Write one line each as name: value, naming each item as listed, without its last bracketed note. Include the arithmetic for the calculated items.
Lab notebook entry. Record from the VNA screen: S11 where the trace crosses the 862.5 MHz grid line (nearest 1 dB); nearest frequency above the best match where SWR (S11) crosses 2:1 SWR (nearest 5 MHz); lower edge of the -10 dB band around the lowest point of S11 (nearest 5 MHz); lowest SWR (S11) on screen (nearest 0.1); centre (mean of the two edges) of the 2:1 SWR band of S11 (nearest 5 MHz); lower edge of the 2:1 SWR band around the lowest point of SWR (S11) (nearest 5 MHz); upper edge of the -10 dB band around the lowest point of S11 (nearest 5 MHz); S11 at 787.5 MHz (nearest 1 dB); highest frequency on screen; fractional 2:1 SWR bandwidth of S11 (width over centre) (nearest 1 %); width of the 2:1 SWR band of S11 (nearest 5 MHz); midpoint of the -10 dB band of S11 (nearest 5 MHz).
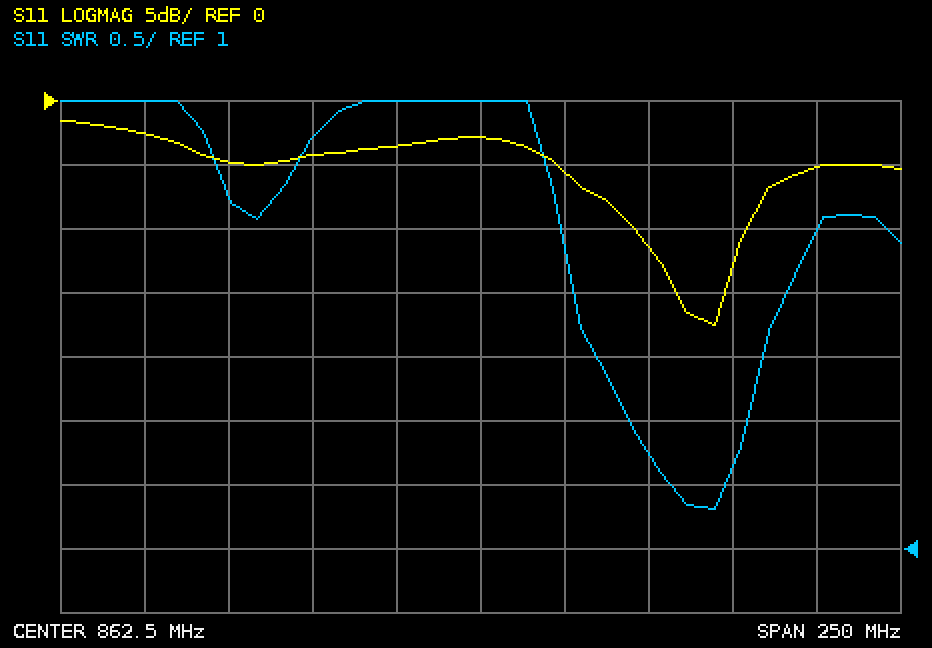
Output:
S11 where the trace crosses the 862.5 MHz grid line: -3 dB
nearest frequency above the best match where SWR (S11) crosses 2:1 SWR: 940 MHz
lower edge of the -10 dB band around the lowest point of S11: 910 MHz
lowest SWR (S11) on screen: 1.3
centre (mean of the two edges) of the 2:1 SWR band of S11: 925 MHz
lower edge of the 2:1 SWR band around the lowest point of SWR (S11): 905 MHz
upper edge of the -10 dB band around the lowest point of S11: 940 MHz
S11 at 787.5 MHz: -5 dB
highest frequency on screen: 987.5 MHz
fractional 2:1 SWR bandwidth of S11 (width over centre): 35 MHz / 922.5 MHz ≈ 4 %
width of the 2:1 SWR band of S11: 940 MHz − 905 MHz = 35 MHz
midpoint of the -10 dB band of S11: 925 MHz
